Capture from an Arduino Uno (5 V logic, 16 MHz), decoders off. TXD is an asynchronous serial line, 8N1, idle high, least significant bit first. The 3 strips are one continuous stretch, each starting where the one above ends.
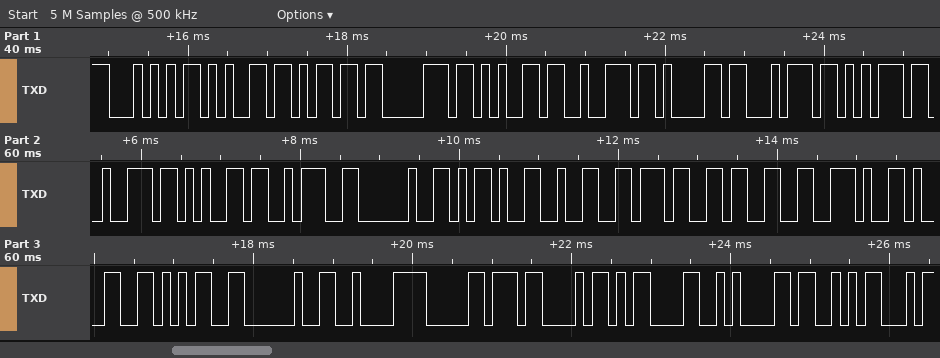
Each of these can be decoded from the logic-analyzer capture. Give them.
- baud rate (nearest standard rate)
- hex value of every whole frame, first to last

9600 baud
54 65 6D 70 65 72 61 74 75 72 65 3A 20 2D 32 37 33 2E 31 35 20 C2 B0 43 0D 0A 53
